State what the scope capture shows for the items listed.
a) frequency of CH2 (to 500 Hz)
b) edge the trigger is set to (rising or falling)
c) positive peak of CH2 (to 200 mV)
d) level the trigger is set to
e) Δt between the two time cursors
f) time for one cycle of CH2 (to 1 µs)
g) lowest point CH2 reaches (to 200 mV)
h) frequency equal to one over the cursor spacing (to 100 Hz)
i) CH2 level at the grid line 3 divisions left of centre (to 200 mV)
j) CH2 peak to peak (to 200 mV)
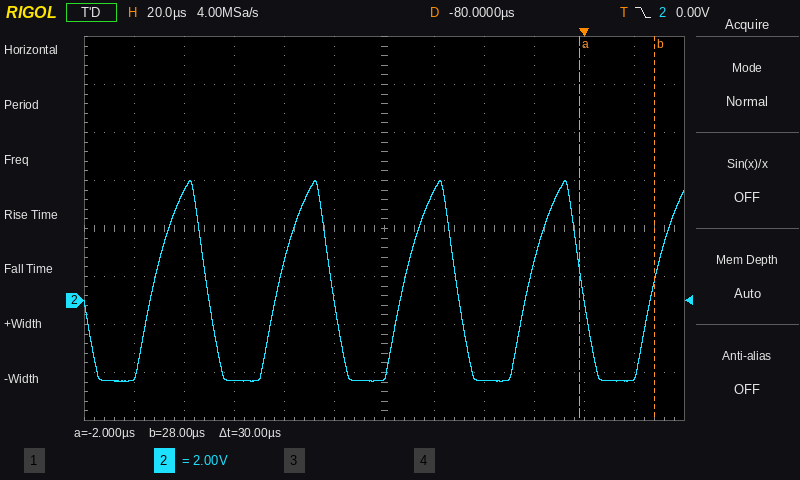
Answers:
20.0 kHz
falling
5.0 V
0.00 V
30 µs
50 µs
-3.4 V
33.3 kHz
-3.4 V
8.4 V
